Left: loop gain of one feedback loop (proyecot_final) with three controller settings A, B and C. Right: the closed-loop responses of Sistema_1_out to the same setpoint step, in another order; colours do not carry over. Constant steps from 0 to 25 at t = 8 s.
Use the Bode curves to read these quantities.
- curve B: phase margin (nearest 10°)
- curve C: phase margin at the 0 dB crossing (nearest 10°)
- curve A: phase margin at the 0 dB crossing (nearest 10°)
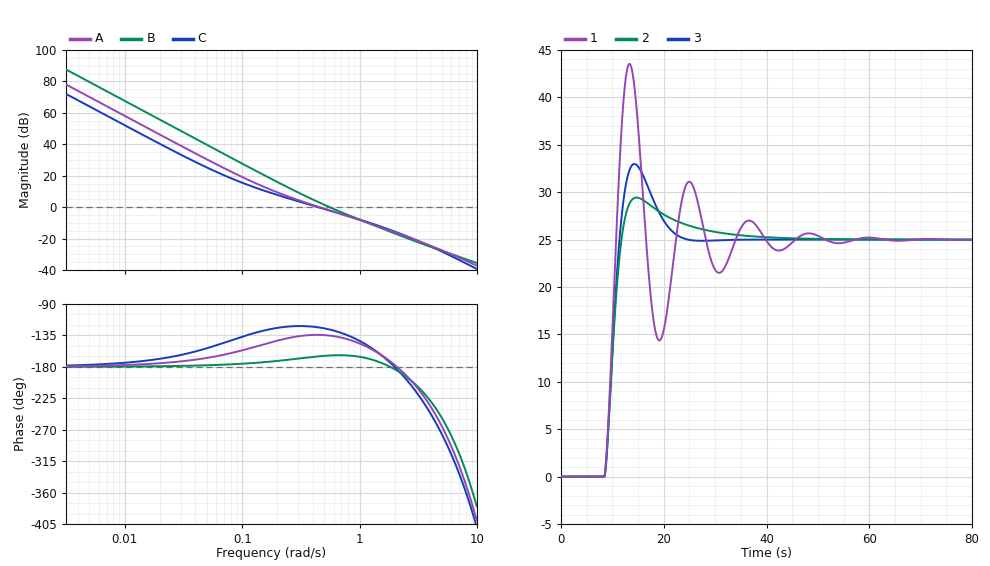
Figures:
20°
60°
50°
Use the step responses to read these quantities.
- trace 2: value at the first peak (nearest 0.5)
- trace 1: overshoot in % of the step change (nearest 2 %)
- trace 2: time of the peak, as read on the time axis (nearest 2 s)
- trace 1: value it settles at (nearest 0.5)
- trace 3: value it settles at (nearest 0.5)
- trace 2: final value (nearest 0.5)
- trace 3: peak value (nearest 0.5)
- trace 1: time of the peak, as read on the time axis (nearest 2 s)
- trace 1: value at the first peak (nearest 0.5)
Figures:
29.5
74 %
14 s
25.0
25.0
25.0
33.0
14 s
43.5
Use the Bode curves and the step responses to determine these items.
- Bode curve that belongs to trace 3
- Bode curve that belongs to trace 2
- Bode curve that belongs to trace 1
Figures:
A
C
B
